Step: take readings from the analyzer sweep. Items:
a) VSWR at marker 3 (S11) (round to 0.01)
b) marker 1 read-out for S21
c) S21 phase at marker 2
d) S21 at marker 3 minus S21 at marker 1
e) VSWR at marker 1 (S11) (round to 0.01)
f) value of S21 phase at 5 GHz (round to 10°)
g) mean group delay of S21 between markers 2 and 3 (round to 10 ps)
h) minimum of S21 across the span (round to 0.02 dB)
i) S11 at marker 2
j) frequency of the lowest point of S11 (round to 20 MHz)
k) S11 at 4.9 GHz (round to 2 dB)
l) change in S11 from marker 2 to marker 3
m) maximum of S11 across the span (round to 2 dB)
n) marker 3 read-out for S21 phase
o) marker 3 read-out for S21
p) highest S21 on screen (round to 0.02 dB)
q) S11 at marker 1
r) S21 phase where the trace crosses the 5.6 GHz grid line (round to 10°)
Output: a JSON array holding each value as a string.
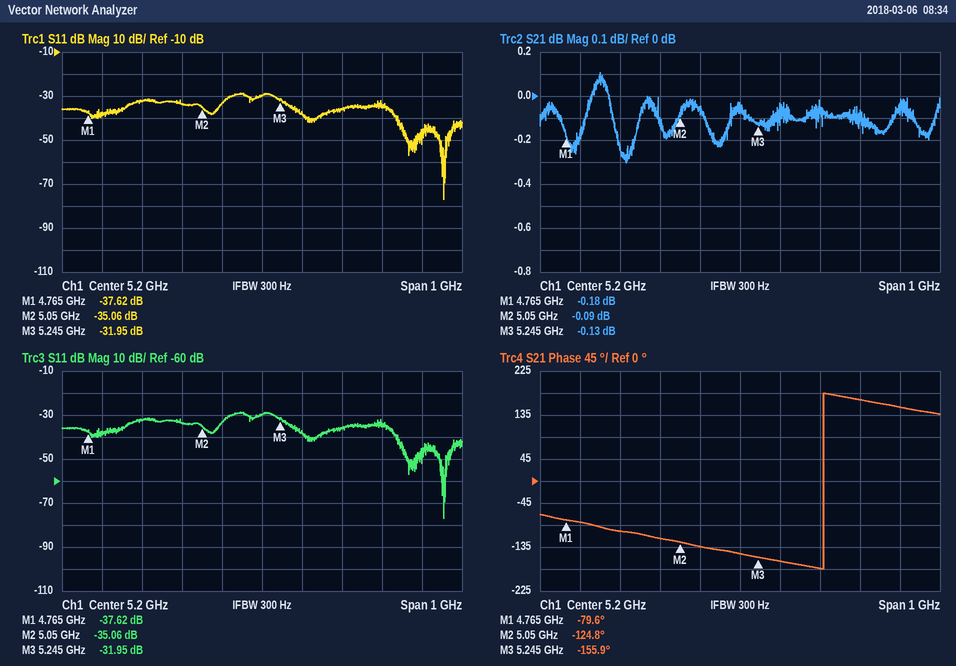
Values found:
["1.05", "-0.18 dB", "-124.8°", "0.05 dB", "1.03", "-120°", "440 ps", "-0.30 dB", "-35.06 dB", "5.66 GHz", "-32 dB", "3.11 dB", "-28 dB", "-155.9°", "-0.13 dB", "0.10 dB", "-37.62 dB", "150°"]
